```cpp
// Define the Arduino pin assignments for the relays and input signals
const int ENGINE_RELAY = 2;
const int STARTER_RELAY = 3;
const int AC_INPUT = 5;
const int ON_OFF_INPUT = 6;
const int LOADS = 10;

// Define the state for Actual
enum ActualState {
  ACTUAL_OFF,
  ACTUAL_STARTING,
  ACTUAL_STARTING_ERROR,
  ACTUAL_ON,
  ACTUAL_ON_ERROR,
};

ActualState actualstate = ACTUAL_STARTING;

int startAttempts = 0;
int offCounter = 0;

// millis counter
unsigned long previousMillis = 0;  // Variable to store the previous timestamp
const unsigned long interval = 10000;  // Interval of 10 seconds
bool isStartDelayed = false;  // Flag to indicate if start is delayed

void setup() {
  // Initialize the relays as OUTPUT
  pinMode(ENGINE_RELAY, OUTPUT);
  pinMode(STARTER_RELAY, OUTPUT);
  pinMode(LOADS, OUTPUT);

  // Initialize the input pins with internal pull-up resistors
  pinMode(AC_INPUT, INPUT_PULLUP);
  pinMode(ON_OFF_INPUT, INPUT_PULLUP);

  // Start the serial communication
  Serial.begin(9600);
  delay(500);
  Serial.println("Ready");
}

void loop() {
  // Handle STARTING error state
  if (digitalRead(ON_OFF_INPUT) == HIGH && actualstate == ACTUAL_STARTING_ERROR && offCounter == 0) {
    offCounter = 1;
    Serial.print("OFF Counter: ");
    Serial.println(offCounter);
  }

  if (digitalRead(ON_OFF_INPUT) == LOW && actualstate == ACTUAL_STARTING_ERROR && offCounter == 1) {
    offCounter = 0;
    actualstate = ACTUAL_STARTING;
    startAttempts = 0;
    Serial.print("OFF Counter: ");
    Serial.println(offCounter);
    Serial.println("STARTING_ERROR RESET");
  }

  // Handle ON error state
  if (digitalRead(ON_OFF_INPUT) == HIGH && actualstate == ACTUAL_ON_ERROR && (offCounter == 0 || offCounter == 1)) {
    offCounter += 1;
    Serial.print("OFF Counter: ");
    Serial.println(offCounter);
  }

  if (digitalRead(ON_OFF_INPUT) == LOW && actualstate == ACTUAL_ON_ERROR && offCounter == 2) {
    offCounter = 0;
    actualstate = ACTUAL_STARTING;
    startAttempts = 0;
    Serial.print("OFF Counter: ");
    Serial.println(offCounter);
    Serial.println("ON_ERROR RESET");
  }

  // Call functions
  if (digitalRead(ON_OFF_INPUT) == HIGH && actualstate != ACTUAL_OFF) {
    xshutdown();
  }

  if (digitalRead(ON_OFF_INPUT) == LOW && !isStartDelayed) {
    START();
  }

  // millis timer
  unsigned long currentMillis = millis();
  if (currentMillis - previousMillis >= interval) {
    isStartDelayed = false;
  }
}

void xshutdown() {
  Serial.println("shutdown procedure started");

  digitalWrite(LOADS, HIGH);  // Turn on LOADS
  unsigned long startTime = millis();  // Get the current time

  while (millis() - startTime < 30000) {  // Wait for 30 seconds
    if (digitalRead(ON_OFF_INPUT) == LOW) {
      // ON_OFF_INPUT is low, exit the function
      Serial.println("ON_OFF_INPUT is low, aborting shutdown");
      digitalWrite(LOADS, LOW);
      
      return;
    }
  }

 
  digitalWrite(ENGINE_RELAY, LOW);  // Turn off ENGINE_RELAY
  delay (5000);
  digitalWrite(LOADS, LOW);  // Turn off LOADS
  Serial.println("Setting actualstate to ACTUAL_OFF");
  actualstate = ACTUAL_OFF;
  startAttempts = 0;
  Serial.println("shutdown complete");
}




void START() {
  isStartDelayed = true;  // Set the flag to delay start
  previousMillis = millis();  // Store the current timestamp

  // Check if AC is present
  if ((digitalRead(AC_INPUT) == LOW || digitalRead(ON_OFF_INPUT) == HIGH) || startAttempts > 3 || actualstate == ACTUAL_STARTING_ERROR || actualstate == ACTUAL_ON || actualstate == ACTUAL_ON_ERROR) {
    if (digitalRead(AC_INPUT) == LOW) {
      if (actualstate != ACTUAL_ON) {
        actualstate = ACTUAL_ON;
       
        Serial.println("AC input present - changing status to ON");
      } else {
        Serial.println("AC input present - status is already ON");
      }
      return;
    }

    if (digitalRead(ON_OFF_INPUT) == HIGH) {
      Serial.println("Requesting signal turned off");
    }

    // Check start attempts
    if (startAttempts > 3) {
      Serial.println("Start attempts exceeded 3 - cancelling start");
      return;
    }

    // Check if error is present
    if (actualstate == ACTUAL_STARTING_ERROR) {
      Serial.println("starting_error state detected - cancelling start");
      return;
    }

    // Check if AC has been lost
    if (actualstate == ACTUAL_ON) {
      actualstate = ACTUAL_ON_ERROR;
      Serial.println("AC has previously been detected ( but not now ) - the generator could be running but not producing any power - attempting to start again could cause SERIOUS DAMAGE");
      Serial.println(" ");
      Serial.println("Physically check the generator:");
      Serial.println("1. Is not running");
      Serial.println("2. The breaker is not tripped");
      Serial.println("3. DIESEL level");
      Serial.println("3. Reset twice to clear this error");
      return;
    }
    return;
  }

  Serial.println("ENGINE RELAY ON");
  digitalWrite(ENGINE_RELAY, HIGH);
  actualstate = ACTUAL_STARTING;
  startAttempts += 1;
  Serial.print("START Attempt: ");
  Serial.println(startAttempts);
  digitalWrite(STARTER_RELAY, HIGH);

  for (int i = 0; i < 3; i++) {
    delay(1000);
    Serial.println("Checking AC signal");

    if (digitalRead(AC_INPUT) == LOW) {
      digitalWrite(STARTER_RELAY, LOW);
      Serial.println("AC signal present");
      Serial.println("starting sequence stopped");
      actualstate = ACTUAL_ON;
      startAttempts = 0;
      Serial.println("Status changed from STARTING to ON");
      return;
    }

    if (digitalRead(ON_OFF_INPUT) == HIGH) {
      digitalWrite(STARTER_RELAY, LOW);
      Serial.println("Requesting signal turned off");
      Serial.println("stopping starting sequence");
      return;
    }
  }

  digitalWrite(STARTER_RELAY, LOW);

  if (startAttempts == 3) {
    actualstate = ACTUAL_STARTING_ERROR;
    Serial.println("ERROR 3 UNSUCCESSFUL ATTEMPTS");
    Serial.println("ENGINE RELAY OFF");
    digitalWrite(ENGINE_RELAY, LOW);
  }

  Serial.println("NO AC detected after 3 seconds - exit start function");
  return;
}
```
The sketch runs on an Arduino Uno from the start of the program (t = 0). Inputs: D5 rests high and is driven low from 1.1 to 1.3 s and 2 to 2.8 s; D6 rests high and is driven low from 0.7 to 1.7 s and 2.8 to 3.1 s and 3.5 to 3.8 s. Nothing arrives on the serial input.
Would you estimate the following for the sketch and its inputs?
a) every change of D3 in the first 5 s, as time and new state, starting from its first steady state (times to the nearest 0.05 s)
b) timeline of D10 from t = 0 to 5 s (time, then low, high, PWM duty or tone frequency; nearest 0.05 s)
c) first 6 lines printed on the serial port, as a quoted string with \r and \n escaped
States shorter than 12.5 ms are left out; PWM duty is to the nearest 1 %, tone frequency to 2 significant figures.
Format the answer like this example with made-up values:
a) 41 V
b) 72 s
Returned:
a) 0 s low; 0.7 s high; 1.7 s low
b) 0 s low; 0.5 s high; 0.7 s low; 1.75 s high; 2.8 s low; 3.1 s high; 3.5 s low; 3.8 s high
c) "Ready\r\nshutdown procedure started\r\nON_OFF_INPUT is low, aborting shutdown\r\nENGINE RELAY ON\r\nSTART Attempt: 1\r\nChecking AC signal\r\n"
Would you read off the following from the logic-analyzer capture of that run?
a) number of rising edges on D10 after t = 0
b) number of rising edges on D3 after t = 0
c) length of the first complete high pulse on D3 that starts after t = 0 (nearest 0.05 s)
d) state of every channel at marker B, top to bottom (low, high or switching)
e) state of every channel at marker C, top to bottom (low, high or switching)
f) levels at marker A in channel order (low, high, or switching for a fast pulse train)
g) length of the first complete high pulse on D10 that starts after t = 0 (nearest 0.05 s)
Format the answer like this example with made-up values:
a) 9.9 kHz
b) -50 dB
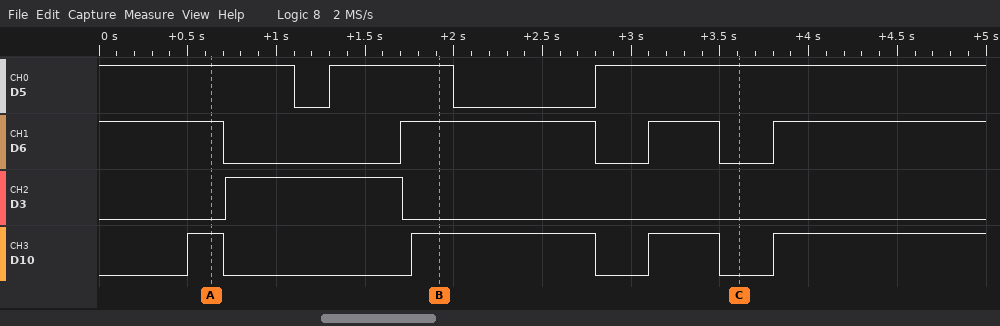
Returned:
a) 4
b) 1
c) 1.00 s
d) D5 high, D6 high, D3 low, D10 high
e) D5 high, D6 low, D3 low, D10 low
f) D5 high, D6 high, D3 low, D10 high
g) 0.20 s
